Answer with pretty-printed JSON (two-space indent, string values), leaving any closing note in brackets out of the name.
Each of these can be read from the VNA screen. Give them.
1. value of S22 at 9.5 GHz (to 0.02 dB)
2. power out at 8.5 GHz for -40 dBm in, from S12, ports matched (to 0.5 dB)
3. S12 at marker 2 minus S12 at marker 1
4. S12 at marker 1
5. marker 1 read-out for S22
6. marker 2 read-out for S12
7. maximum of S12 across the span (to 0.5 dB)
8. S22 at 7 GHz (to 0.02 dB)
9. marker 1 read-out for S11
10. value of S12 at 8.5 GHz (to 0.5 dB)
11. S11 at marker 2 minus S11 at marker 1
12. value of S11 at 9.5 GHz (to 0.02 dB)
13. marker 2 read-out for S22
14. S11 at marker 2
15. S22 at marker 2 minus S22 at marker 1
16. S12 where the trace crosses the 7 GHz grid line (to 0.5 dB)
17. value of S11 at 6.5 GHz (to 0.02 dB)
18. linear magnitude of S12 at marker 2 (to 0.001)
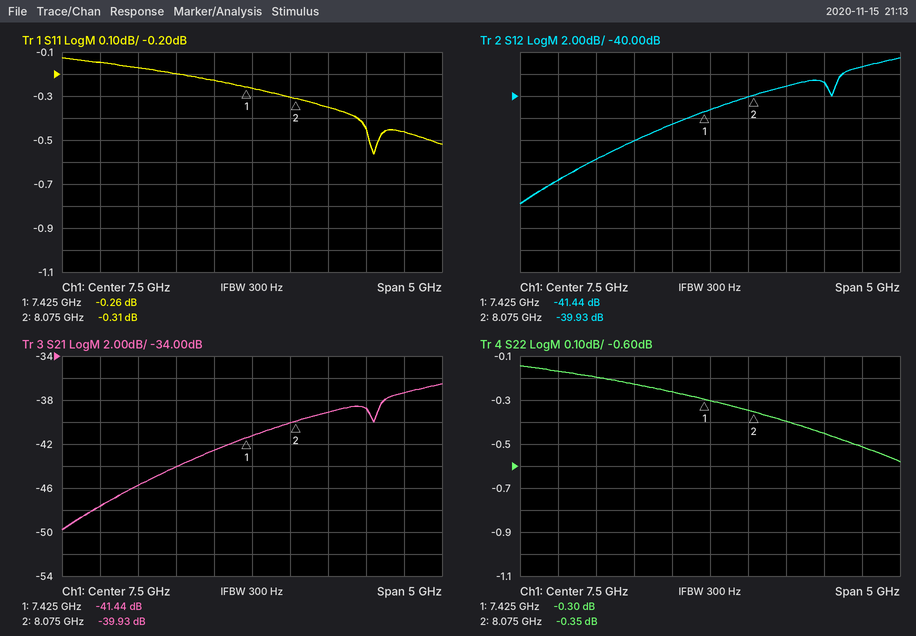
{
  "value of S22 at 9.5 GHz": "-0.52 dB",
  "power out at 8.5 GHz for -40 dBm in, from S12, ports matched": "-79.0 dBm",
  "S12 at marker 2 minus S12 at marker 1": "1.51 dB",
  "S12 at marker 1": "-41.44 dB",
  "marker 1 read-out for S22": "-0.30 dB",
  "marker 2 read-out for S12": "-39.93 dB",
  "maximum of S12 across the span": "-36.5 dB",
  "S22 at 7 GHz": "-0.26 dB",
  "marker 1 read-out for S11": "-0.26 dB",
  "value of S12 at 8.5 GHz": "-39.0 dB",
  "S11 at marker 2 minus S11 at marker 1": "-0.05 dB",
  "value of S11 at 9.5 GHz": "-0.46 dB",
  "marker 2 read-out for S22": "-0.35 dB",
  "S11 at marker 2": "-0.31 dB",
  "S22 at marker 2 minus S22 at marker 1": "-0.05 dB",
  "S12 where the trace crosses the 7 GHz grid line": "-42.5 dB",
  "value of S11 at 6.5 GHz": "-0.20 dB",
  "linear magnitude of S12 at marker 2": "0.010"
}
